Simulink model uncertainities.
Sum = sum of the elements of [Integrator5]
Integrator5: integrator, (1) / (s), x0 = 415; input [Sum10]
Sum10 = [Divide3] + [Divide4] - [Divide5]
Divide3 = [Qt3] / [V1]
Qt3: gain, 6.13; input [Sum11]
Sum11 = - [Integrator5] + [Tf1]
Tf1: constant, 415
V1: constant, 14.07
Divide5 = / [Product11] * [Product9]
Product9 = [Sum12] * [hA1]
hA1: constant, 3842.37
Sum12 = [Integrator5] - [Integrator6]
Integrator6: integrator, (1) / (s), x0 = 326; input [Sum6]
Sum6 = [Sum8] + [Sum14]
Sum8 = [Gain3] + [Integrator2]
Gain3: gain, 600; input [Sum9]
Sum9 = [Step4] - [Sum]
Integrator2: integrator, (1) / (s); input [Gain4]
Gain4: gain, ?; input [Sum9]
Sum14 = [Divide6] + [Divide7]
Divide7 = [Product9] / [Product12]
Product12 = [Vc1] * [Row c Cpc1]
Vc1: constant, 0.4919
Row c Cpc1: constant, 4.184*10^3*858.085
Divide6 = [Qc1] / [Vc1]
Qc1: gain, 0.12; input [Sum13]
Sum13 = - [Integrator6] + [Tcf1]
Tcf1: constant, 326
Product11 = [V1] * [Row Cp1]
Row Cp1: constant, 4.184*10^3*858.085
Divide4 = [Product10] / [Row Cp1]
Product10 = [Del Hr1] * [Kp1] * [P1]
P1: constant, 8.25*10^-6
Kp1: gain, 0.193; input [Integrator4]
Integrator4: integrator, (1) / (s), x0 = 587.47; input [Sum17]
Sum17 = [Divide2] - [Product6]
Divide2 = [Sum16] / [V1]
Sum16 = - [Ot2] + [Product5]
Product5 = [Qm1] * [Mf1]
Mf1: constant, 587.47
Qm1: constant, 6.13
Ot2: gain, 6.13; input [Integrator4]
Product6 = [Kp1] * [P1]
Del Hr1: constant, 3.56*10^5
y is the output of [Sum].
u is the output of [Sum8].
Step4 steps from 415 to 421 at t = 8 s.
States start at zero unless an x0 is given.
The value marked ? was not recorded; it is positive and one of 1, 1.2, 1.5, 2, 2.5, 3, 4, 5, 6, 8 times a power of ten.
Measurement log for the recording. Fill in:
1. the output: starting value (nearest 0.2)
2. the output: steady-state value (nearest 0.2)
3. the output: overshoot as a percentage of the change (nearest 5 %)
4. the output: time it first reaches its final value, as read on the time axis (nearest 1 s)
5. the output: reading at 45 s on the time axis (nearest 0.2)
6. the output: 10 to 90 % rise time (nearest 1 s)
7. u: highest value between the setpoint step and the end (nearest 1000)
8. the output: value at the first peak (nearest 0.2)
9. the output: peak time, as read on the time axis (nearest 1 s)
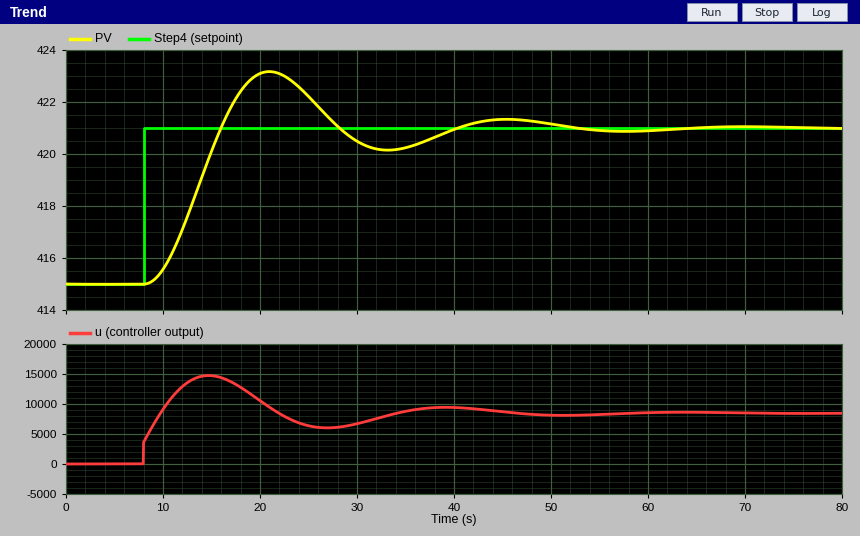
415.0
421.0
35 %
16 s
421.4
5 s
15000
423.2
21 s
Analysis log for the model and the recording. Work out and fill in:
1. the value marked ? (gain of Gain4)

500
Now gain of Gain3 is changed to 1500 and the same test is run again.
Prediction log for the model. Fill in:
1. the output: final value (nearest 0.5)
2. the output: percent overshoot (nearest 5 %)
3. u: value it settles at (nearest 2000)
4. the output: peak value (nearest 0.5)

421.0
20 %
8000
422.0
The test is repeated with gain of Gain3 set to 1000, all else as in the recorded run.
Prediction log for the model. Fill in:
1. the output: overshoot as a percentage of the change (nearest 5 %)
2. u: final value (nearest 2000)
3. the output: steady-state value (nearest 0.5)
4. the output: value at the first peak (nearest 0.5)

25 %
8000
421.0
422.5
